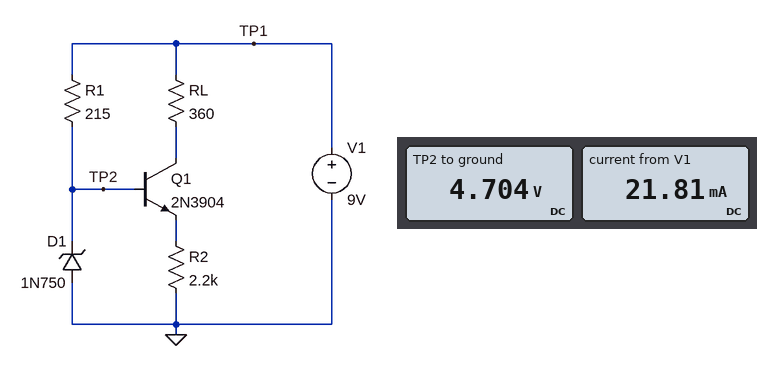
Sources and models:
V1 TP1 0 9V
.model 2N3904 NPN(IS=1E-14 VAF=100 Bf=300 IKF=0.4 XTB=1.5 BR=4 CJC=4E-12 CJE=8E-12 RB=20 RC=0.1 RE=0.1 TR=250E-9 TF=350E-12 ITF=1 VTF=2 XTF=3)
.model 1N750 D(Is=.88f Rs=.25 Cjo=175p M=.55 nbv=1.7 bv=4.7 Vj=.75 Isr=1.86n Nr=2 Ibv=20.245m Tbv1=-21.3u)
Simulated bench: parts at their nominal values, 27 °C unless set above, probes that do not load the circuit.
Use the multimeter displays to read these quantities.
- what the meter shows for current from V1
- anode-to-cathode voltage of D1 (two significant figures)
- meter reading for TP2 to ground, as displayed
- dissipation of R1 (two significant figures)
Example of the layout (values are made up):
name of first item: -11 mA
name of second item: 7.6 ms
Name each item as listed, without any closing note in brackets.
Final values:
what the meter shows for current from V1: 21.81 mA
anode-to-cathode voltage of D1: -4.7 V
meter reading for TP2 to ground, as displayed: 4.704 V
dissipation of R1: 86 mW
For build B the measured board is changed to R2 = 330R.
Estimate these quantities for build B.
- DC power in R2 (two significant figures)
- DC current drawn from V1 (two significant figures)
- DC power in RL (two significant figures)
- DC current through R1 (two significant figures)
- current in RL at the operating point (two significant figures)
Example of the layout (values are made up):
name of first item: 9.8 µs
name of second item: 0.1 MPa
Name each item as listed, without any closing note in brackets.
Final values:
DC power in R2: 48 mW
DC current drawn from V1: 32 mA
DC power in RL: 52 mW
DC current through R1: 20 mA
current in RL at the operating point: 12 mA
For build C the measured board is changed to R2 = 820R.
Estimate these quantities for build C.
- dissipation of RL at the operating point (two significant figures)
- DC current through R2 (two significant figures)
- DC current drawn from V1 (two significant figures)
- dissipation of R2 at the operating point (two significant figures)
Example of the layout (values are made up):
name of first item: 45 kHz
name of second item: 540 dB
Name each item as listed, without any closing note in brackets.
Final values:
dissipation of RL at the operating point: 8.5 mW
DC current through R2: 4.9 mA
DC current drawn from V1: 25 mA
dissipation of R2 at the operating point: 20 mW
